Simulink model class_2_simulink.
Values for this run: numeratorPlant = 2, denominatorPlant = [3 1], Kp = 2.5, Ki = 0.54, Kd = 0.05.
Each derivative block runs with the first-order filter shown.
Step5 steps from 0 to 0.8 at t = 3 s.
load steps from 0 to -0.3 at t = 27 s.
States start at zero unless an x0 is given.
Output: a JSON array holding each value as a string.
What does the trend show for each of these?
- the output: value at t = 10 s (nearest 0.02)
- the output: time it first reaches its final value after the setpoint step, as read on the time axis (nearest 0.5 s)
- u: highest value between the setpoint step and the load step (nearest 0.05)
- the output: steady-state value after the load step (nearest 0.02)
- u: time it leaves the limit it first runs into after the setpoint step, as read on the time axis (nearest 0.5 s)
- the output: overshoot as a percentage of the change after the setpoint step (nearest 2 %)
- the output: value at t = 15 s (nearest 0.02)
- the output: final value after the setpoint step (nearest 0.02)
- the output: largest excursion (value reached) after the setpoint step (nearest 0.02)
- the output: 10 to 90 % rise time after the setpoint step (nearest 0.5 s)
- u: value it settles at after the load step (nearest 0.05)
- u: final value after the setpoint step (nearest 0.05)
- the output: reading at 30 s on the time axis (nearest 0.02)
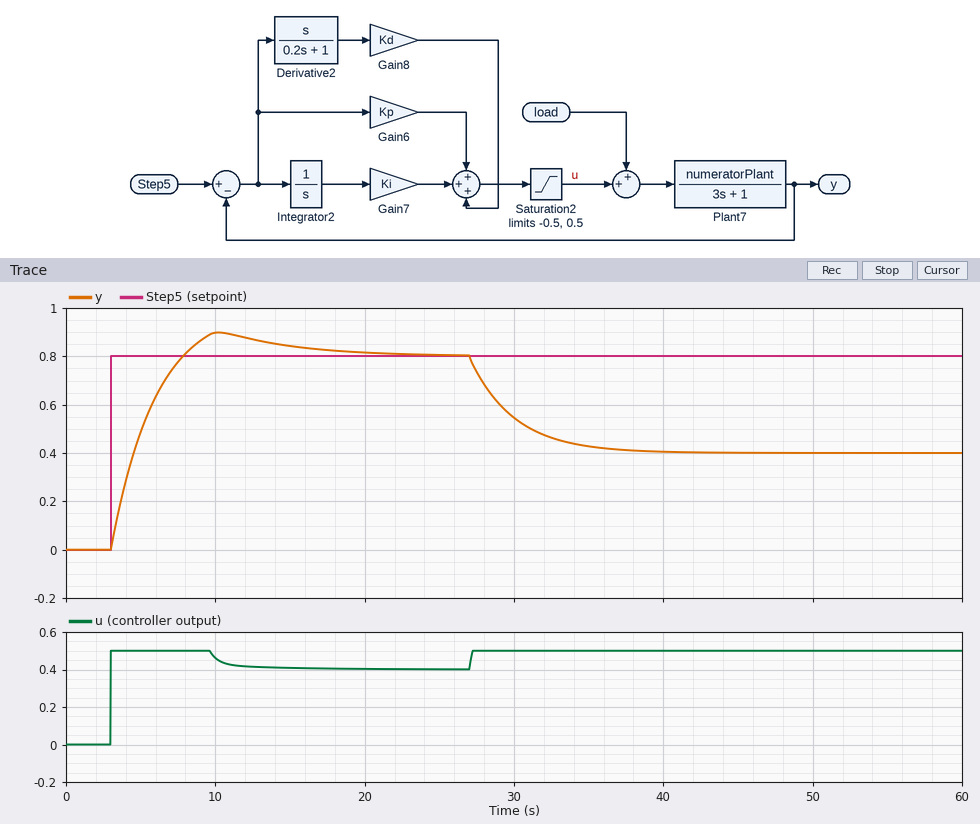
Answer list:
["0.90", "8.0 s", "0.50", "0.40", "9.5 s", "12 %", "0.84", "0.80", "0.90", "3.5 s", "0.50", "0.40", "0.54"]
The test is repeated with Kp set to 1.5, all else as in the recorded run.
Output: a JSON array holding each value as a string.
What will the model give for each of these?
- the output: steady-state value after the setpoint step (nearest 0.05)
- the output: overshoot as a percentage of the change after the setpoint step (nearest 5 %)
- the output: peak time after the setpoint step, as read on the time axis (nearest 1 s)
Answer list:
["0.80", "15 %", "11 s"]
